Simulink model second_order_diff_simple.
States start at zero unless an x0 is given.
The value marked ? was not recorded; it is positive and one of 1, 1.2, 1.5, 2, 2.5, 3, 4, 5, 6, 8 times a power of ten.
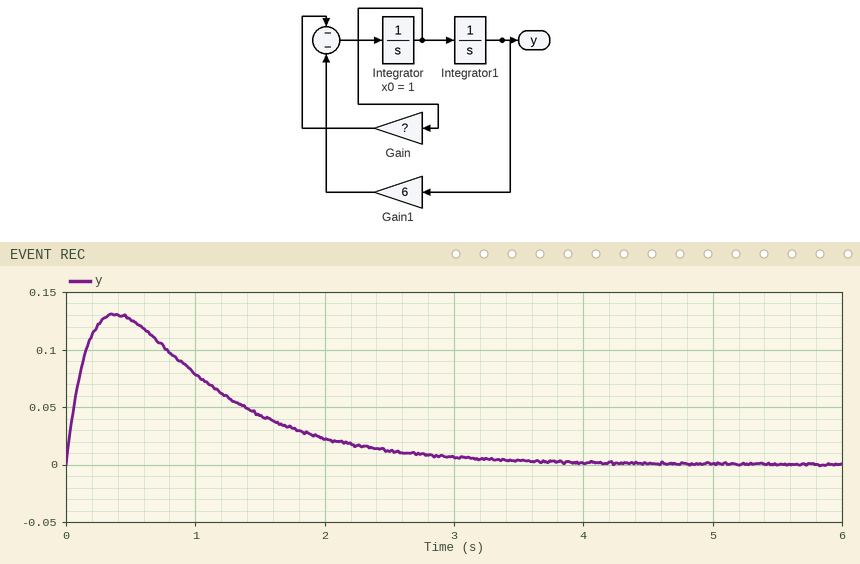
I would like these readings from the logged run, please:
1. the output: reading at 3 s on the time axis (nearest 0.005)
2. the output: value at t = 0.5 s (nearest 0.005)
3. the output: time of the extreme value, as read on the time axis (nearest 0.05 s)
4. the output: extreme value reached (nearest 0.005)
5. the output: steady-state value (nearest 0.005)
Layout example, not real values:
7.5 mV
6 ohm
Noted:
0.005
0.125
0.40 s
0.130
0.000
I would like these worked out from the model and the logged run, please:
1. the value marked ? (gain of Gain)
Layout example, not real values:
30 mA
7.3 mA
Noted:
6
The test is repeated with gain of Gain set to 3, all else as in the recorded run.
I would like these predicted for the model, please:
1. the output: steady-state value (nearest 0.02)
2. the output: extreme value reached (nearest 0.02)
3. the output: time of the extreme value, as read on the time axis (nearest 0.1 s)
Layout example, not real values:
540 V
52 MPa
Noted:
0.00
0.20
0.5 s
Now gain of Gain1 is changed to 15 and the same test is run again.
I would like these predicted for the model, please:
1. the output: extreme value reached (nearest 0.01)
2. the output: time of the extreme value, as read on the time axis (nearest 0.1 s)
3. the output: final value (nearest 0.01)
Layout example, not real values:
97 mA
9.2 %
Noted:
0.11
0.3 s
0.00
